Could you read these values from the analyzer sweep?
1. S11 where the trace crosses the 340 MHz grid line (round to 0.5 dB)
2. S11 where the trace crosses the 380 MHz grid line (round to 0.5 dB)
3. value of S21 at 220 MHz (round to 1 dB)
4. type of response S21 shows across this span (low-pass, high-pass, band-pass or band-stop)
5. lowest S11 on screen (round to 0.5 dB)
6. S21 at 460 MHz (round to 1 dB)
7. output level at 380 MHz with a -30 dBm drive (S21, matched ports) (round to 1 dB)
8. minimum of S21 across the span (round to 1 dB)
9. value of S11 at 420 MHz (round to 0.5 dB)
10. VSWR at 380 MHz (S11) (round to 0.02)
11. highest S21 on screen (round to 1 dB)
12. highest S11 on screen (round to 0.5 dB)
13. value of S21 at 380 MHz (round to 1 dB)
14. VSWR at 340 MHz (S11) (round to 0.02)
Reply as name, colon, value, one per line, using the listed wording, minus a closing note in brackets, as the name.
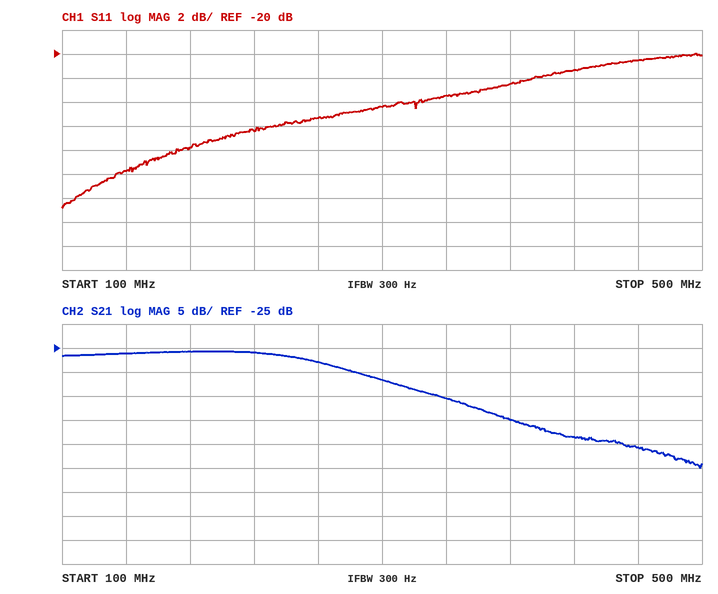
S11 where the trace crosses the 340 MHz grid line: -23.5 dB
S11 where the trace crosses the 380 MHz grid line: -22.5 dB
value of S21 at 220 MHz: -26 dB
type of response S21 shows across this span: low-pass
lowest S11 on screen: -33.0 dB
S21 at 460 MHz: -46 dB
output level at 380 MHz with a -30 dBm drive (S21, matched ports): -70 dBm
minimum of S21 across the span: -50 dB
value of S11 at 420 MHz: -21.5 dB
VSWR at 380 MHz (S11): 1.16
highest S21 on screen: -26 dB
highest S11 on screen: -20.0 dB
value of S21 at 380 MHz: -40 dB
VSWR at 340 MHz (S11): 1.14
